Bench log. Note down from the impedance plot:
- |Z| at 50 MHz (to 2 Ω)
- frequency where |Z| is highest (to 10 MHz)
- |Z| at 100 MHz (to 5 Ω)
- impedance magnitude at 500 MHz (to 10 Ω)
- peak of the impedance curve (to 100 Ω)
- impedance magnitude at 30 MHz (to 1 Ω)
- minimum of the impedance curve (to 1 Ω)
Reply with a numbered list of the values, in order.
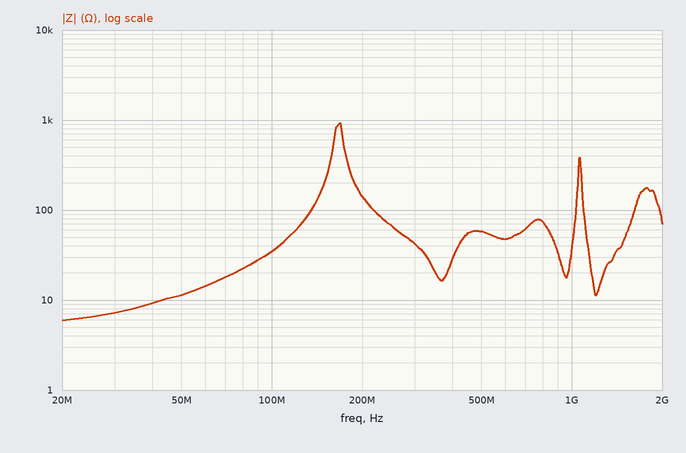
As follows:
1. 12 Ω
2. 170 MHz
3. 35 Ω
4. 60 Ω
5. 900 Ω
6. 7 Ω
7. 6 Ω
